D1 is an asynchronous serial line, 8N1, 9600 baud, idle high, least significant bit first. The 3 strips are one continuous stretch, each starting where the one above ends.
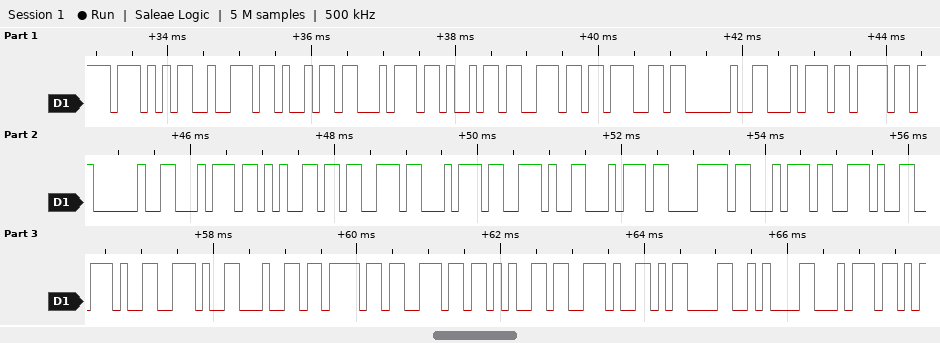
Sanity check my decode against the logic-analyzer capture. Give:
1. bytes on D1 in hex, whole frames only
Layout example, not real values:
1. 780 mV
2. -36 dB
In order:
1. 0x57 0x72 0x69 0x74 0x69 0x6E 0x67 0x20 0x74 0x6F 0x20 0x74 0x65 0x73 0x74 0x2E 0x74 0x78 0x74 0x2E 0x2E 0x2E 0x64 0x6F 0x6E 0x65 0x2E 0x0D 0x0A 0x74
